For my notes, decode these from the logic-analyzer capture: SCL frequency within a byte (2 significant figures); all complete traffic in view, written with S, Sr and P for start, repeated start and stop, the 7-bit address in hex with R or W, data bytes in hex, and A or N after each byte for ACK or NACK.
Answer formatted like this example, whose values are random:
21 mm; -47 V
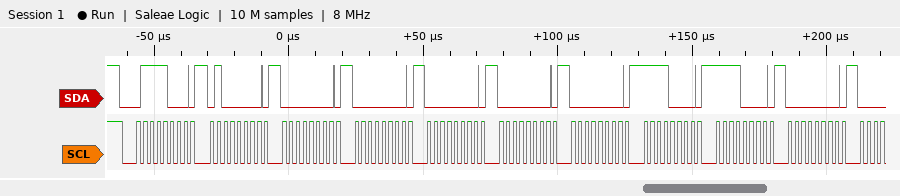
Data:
400 kHz; S 3CW A 40 A 00 A 00 A 00 A 00 A 00 A F0 A F0 A 00 A
